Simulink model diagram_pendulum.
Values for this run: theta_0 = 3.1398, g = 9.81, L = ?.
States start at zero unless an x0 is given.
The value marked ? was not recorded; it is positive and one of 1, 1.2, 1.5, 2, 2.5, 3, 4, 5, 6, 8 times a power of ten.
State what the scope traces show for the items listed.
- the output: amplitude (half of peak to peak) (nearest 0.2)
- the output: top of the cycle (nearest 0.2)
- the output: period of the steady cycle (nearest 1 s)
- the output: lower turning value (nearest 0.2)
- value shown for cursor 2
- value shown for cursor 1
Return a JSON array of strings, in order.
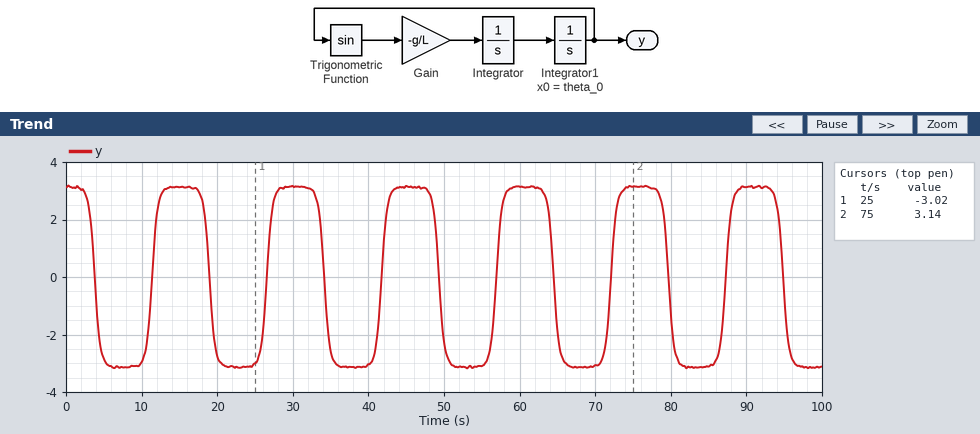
["3.2", "3.2", "15 s", "-3.2", "3.14", "-3.02"]
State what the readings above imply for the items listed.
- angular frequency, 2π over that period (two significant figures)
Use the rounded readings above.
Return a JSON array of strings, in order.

["0.42 rad/s"]
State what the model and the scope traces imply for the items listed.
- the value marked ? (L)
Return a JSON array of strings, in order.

["2"]
